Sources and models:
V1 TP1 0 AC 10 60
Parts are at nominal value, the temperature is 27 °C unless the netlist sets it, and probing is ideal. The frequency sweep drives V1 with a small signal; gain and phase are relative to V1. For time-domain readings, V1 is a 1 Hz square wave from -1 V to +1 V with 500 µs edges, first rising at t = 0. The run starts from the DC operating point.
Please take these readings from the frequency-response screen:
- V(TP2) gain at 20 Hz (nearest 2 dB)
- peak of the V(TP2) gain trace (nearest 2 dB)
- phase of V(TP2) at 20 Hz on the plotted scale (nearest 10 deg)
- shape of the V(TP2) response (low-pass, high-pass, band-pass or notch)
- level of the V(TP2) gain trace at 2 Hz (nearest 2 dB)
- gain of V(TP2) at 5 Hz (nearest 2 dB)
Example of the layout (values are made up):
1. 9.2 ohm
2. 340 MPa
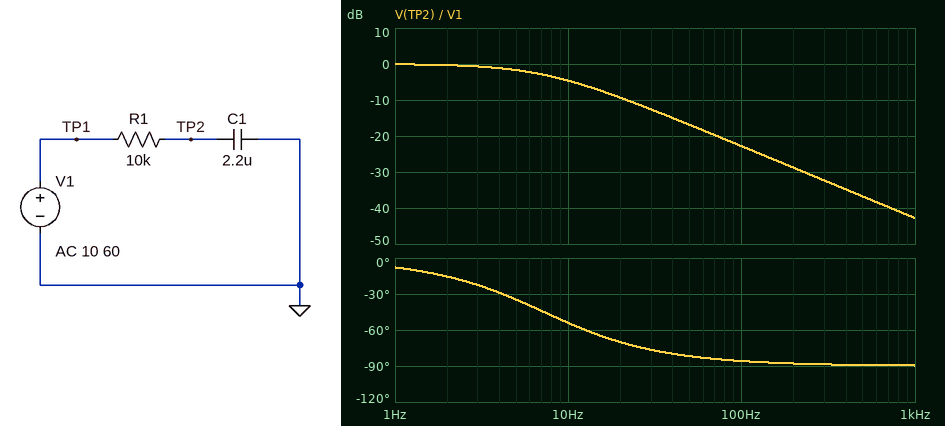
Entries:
1. -10 dB
2. 0 dB
3. -70 deg
4. low-pass
5. 0 dB
6. -2 dB
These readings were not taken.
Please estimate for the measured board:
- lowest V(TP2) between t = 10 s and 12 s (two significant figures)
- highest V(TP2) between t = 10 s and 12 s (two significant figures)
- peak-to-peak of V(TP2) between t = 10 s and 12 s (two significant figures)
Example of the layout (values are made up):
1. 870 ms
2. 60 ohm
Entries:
1. -1.0 V
2. 1.0 V
3. 2.0 V
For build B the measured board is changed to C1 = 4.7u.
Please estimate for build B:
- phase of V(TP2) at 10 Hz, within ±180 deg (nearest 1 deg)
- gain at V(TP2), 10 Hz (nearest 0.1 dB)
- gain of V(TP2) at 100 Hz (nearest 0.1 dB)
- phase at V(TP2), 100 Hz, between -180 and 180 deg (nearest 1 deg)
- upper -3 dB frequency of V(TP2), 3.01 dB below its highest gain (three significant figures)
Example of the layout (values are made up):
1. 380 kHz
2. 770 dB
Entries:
1. -71 deg
2. -9.9 dB
3. -29.4 dB
4. -88 deg
5. 3.39 Hz
